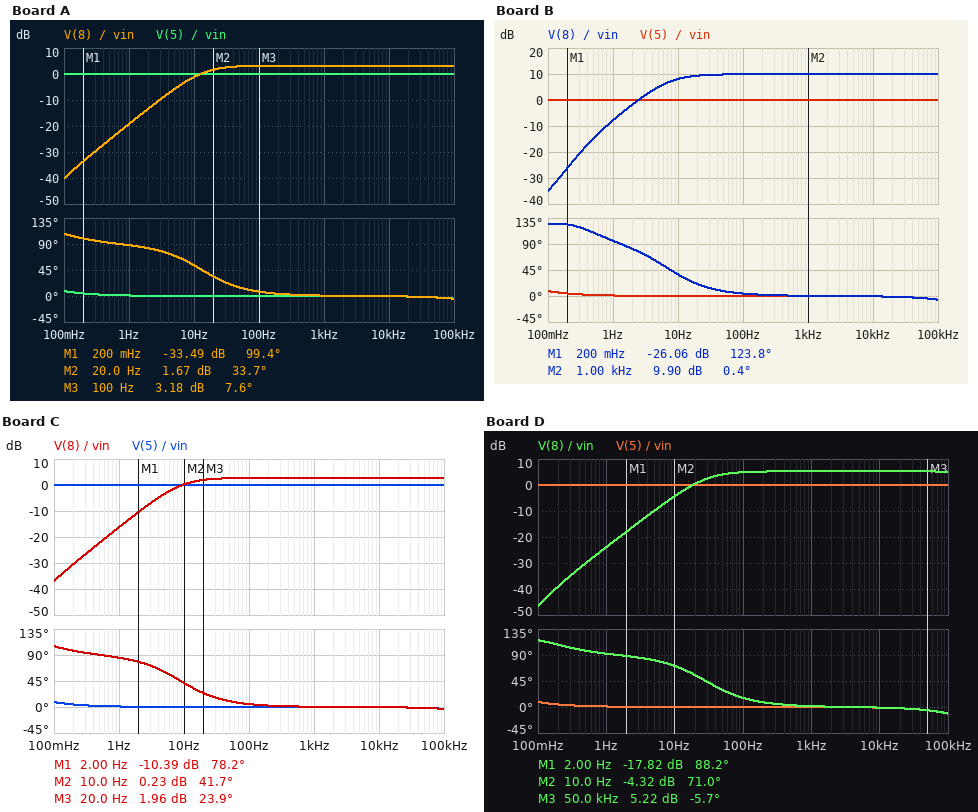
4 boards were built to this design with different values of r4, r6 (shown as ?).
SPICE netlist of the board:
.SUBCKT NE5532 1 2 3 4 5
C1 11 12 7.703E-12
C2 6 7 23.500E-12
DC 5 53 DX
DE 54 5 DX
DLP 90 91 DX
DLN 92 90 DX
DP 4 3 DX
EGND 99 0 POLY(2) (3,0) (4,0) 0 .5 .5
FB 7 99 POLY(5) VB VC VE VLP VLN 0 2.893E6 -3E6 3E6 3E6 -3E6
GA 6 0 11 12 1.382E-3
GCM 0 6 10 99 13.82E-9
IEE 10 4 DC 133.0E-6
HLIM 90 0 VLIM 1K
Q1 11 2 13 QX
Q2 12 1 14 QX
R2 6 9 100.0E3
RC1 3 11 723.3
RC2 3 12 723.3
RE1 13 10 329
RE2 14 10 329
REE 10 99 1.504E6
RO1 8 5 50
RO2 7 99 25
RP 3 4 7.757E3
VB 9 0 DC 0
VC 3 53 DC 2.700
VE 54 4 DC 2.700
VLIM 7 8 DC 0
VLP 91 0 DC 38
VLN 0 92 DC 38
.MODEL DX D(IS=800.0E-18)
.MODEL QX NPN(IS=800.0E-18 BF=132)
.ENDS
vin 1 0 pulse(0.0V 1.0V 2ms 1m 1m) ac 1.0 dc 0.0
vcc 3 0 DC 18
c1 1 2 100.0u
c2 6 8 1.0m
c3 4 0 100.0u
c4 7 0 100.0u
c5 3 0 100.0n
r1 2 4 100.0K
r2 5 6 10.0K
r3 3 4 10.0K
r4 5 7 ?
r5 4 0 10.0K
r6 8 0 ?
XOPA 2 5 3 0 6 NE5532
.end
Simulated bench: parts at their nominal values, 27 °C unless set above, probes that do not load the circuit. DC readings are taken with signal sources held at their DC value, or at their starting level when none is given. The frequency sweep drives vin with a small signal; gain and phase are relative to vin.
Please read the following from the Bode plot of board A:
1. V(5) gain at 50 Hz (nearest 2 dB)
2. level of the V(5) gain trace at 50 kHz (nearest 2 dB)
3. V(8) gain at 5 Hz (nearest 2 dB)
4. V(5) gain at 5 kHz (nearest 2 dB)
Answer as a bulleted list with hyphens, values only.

- 0 dB
- 0 dB
- -6 dB
- 0 dB
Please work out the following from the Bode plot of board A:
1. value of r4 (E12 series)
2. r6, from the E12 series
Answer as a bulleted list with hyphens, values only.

- 22 kΩ
- 12 Ω
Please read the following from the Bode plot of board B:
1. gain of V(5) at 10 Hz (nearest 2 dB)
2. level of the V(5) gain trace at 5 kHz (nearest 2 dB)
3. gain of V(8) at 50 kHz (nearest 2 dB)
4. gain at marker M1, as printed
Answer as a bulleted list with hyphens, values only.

- 0 dB
- 0 dB
- 10 dB
- -26.06 dB
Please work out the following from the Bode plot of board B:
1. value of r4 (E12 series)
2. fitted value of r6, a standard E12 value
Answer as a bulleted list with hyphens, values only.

- 4.7 kΩ
- 22 Ω
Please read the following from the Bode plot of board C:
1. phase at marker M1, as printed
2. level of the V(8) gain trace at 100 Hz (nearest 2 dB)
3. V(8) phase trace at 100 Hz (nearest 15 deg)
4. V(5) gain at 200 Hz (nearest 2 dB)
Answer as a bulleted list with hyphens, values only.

- 78.2 deg
- 2 dB
- 0 deg
- 0 dB
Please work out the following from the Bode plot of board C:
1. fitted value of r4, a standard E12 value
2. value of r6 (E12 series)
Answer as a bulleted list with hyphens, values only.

- 27 kΩ
- 18 Ω
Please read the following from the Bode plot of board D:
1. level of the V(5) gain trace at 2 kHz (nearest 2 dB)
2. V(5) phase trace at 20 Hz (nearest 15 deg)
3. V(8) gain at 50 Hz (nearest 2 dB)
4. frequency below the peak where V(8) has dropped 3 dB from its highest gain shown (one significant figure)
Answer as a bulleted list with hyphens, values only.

- 0 dB
- 0 deg
- 4 dB
- 30 Hz
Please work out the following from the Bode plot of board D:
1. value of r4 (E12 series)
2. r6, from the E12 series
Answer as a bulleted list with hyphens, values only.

- 12 kΩ
- 5.6 Ω
